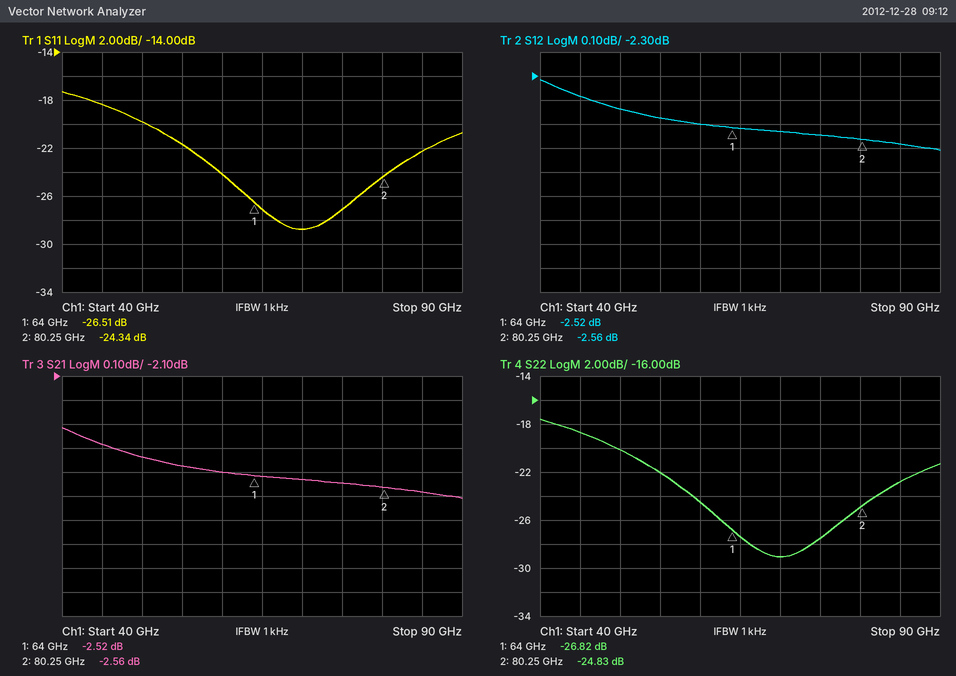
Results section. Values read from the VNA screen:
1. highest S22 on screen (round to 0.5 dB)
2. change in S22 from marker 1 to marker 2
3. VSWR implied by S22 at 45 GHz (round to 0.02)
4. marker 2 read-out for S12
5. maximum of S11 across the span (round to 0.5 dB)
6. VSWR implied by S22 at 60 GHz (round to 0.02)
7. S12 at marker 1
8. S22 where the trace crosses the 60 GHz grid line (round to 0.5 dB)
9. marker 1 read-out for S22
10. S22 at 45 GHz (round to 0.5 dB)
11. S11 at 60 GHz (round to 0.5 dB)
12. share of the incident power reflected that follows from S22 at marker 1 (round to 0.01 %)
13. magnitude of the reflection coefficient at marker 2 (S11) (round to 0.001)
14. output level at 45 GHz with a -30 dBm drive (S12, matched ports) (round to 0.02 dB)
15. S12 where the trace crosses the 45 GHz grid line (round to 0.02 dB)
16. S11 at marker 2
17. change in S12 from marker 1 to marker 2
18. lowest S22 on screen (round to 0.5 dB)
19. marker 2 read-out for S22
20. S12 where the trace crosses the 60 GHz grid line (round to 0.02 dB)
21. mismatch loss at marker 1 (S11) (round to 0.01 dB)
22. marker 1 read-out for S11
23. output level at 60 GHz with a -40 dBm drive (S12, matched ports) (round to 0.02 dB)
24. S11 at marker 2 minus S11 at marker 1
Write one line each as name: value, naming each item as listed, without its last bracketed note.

highest S22 on screen: -17.5 dB
change in S22 from marker 1 to marker 2: 1.99 dB
VSWR implied by S22 at 45 GHz: 1.26
marker 2 read-out for S12: -2.56 dB
maximum of S11 across the span: -17.5 dB
VSWR implied by S22 at 60 GHz: 1.12
S12 at marker 1: -2.52 dB
S22 where the trace crosses the 60 GHz grid line: -24.5 dB
marker 1 read-out for S22: -26.82 dB
S22 at 45 GHz: -18.5 dB
S11 at 60 GHz: -24.0 dB
share of the incident power reflected that follows from S22 at marker 1: 0.21 %
magnitude of the reflection coefficient at marker 2 (S11): 0.061
output level at 45 GHz with a -30 dBm drive (S12, matched ports): -32.38 dBm
S12 where the trace crosses the 45 GHz grid line: -2.38 dB
S11 at marker 2: -24.34 dB
change in S12 from marker 1 to marker 2: -0.04 dB
lowest S22 on screen: -29.0 dB
marker 2 read-out for S22: -24.83 dB
S12 where the trace crosses the 60 GHz grid line: -2.50 dB
mismatch loss at marker 1 (S11): 0.01 dB
marker 1 read-out for S11: -26.51 dB
output level at 60 GHz with a -40 dBm drive (S12, matched ports): -42.50 dBm
S11 at marker 2 minus S11 at marker 1: 2.17 dB
